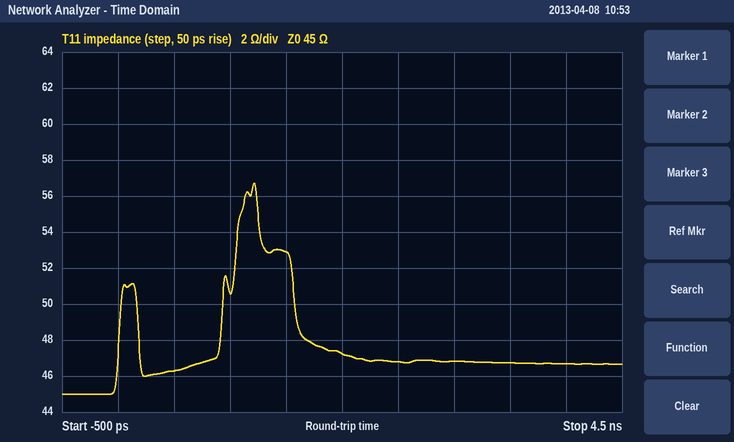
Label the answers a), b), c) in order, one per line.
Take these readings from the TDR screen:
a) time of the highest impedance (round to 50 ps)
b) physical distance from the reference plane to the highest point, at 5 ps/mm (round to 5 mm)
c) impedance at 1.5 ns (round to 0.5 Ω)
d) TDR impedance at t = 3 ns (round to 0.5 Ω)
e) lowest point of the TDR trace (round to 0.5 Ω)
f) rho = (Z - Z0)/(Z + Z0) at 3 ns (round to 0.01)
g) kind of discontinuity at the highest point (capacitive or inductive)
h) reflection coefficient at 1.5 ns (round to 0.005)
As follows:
a) 1.20 ns
b) 120 mm
c) 53.0 Ω
d) 47.0 Ω
e) 45.0 Ω
f) +0.02
g) inductive
h) +0.080
